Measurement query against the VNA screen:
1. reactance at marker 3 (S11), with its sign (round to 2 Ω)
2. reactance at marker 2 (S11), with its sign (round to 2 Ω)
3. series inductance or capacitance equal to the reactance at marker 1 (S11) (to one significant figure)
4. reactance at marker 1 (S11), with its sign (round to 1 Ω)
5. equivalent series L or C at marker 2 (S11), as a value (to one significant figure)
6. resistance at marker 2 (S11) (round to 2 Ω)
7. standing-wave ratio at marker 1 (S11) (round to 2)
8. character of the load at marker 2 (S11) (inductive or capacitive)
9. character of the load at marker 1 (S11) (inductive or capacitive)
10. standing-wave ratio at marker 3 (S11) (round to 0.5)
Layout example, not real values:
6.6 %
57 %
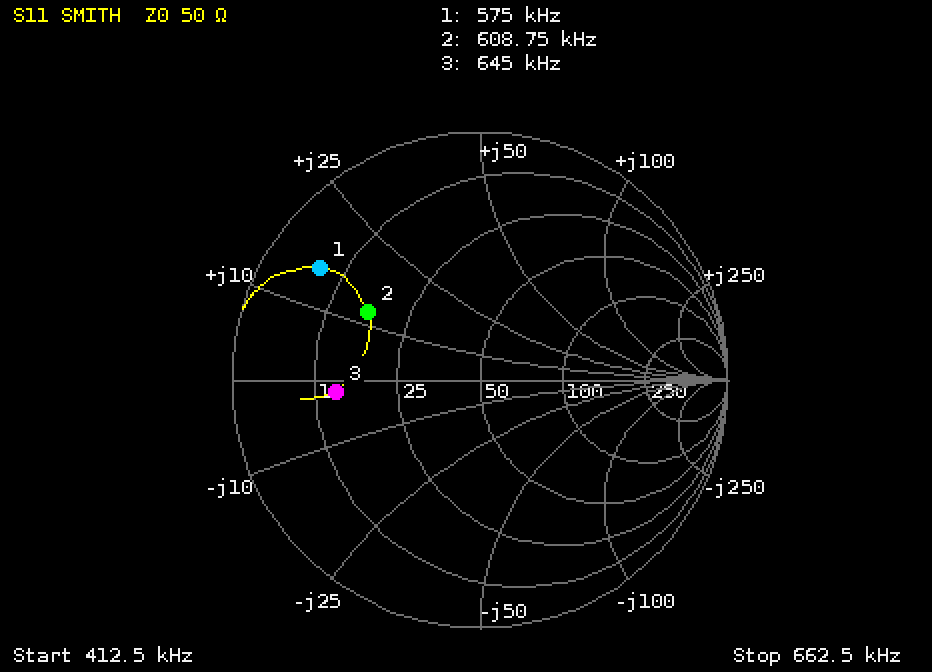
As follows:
-2 Ω
+12 Ω
4 µH
+16 Ω
3 µH
16 Ω
8
inductive
inductive
4.0
